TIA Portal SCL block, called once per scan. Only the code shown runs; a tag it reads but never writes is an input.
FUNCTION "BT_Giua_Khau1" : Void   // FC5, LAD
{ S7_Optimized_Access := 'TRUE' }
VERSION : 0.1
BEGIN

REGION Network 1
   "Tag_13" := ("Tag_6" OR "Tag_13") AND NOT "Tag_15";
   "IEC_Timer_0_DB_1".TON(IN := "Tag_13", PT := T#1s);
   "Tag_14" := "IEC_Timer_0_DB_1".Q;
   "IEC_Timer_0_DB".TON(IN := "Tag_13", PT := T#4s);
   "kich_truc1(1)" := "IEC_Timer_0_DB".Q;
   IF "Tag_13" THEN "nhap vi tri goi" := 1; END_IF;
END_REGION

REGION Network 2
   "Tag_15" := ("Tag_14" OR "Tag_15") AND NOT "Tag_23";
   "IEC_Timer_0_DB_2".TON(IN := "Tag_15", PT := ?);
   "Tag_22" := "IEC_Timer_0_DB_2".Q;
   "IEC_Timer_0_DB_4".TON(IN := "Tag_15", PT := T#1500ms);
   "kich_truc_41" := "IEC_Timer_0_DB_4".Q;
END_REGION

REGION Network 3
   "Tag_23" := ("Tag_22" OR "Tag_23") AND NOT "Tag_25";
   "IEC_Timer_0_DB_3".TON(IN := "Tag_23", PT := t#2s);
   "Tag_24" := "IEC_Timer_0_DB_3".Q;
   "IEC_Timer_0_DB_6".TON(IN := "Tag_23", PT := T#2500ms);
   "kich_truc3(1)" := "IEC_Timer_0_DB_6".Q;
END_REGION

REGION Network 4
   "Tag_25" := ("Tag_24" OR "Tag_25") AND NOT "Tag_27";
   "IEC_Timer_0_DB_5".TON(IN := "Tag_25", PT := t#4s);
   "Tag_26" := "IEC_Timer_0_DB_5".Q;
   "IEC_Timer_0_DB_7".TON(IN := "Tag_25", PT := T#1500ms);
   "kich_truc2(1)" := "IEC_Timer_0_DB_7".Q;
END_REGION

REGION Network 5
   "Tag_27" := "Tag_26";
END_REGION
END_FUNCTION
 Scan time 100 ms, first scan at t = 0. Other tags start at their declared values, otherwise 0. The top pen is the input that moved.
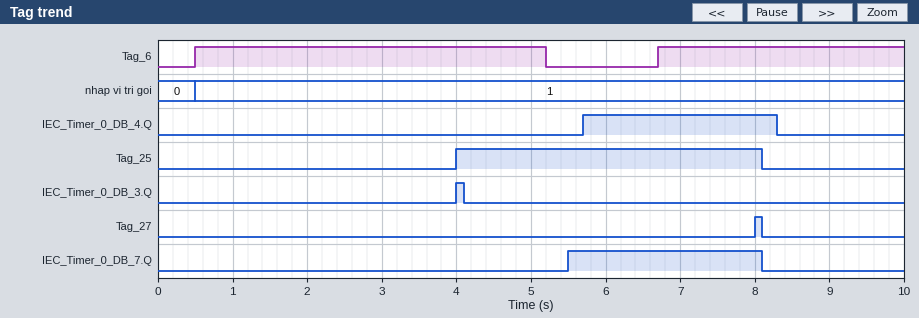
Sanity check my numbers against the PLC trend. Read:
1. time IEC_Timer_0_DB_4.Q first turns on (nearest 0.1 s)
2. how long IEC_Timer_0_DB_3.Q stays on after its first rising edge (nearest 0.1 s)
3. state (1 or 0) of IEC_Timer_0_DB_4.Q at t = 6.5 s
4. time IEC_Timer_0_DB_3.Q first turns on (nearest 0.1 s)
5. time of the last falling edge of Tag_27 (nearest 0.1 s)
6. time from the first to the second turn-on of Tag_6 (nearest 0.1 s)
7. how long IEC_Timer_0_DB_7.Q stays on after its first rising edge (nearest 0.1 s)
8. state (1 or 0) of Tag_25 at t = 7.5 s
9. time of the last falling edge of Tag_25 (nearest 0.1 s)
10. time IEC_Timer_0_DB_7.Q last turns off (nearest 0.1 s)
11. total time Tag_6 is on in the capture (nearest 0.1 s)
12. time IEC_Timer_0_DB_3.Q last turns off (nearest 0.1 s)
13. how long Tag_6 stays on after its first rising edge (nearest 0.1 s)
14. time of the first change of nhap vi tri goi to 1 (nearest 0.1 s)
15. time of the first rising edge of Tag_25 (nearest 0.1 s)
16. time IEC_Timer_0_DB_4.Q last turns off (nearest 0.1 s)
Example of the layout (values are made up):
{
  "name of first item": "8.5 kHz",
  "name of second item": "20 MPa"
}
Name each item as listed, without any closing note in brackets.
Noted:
{
  "time IEC_Timer_0_DB_4.Q first turns on": "5.7 s",
  "how long IEC_Timer_0_DB_3.Q stays on after its first rising edge": "0.1 s",
  "state (1 or 0) of IEC_Timer_0_DB_4.Q at t = 6.5 s": "1",
  "time IEC_Timer_0_DB_3.Q first turns on": "4.0 s",
  "time of the last falling edge of Tag_27": "8.1 s",
  "time from the first to the second turn-on of Tag_6": "6.2 s",
  "how long IEC_Timer_0_DB_7.Q stays on after its first rising edge": "2.6 s",
  "state (1 or 0) of Tag_25 at t = 7.5 s": "1",
  "time of the last falling edge of Tag_25": "8.1 s",
  "time IEC_Timer_0_DB_7.Q last turns off": "8.1 s",
  "total time Tag_6 is on in the capture": "8.0 s",
  "time IEC_Timer_0_DB_3.Q last turns off": "4.1 s",
  "how long Tag_6 stays on after its first rising edge": "4.7 s",
  "time of the first change of nhap vi tri goi to 1": "0.5 s",
  "time of the first rising edge of Tag_25": "4.0 s",
  "time IEC_Timer_0_DB_4.Q last turns off": "8.3 s"
}
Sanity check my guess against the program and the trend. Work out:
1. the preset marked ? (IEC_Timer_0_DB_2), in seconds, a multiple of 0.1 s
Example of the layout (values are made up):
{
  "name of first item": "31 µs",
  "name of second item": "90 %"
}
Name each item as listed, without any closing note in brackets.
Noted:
{
  "the preset marked ? (IEC_Timer_0_DB_2), in seconds, a multiple of 0.1 s": "0.5 s"
}
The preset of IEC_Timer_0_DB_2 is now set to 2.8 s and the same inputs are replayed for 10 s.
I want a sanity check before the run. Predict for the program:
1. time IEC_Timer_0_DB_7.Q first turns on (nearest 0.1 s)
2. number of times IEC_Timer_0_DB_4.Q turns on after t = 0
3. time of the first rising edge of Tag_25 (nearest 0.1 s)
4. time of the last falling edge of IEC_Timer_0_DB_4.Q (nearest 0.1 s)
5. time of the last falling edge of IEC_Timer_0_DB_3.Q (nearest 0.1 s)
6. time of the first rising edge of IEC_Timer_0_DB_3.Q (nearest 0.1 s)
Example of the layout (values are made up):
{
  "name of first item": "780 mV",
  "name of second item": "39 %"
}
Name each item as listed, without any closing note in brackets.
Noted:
{
  "time IEC_Timer_0_DB_7.Q first turns on": "7.8 s",
  "number of times IEC_Timer_0_DB_4.Q turns on after t = 0": "2",
  "time of the first rising edge of Tag_25": "6.3 s",
  "time of the last falling edge of IEC_Timer_0_DB_4.Q": "4.4 s",
  "time of the last falling edge of IEC_Timer_0_DB_3.Q": "6.4 s",
  "time of the first rising edge of IEC_Timer_0_DB_3.Q": "6.3 s"
}
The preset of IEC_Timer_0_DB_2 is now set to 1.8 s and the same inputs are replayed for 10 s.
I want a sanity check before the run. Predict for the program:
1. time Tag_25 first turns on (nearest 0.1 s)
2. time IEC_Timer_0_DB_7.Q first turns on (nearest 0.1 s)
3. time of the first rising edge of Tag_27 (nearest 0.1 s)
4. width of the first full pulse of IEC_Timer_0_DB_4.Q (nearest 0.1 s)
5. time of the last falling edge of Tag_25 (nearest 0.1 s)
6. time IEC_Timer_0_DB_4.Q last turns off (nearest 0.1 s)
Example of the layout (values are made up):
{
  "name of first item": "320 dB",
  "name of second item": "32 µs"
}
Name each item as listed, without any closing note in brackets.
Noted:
{
  "time Tag_25 first turns on": "5.3 s",
  "time IEC_Timer_0_DB_7.Q first turns on": "6.8 s",
  "time of the first rising edge of Tag_27": "9.3 s",
  "width of the first full pulse of IEC_Timer_0_DB_4.Q": "0.4 s",
  "time of the last falling edge of Tag_25": "9.4 s",
  "time IEC_Timer_0_DB_4.Q last turns off": "9.6 s"
}
